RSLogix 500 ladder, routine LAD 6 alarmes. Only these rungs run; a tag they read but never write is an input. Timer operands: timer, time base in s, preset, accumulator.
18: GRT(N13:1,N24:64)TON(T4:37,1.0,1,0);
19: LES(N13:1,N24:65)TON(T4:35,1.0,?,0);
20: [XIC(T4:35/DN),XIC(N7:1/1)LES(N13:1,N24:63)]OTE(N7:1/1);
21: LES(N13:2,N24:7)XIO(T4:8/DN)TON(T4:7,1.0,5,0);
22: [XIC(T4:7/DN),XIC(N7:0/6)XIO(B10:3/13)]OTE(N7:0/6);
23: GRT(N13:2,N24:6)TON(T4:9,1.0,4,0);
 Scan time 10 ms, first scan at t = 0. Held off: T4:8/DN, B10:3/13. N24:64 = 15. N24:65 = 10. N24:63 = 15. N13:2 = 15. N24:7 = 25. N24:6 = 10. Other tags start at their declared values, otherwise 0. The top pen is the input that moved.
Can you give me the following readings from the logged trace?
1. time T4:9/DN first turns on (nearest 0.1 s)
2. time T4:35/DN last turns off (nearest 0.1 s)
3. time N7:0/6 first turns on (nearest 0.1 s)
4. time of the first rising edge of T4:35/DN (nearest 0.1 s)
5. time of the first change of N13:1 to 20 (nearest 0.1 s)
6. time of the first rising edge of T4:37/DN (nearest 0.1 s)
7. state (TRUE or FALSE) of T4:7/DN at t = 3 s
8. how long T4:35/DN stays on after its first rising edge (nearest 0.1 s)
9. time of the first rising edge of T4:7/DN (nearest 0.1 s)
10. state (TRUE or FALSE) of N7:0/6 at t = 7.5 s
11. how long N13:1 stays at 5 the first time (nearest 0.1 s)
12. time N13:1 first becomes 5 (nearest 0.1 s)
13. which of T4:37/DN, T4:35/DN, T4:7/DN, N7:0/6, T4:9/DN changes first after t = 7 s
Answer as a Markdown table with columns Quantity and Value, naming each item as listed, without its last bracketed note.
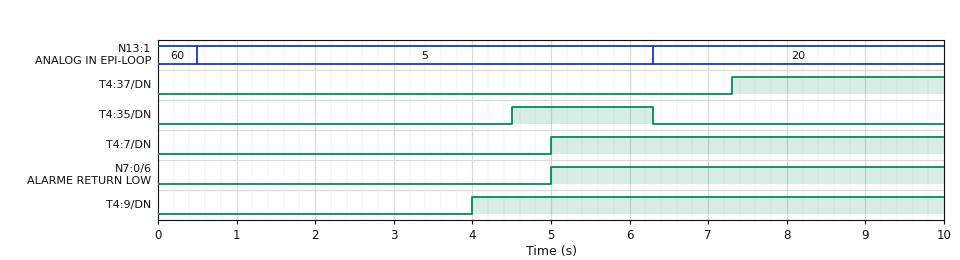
| Quantity | Value |
|---|---|
| time T4:9/DN first turns on | 4.0 s |
| time T4:35/DN last turns off | 6.3 s |
| time N7:0/6 first turns on | 5.0 s |
| time of the first rising edge of T4:35/DN | 4.5 s |
| time of the first change of N13:1 to 20 | 6.3 s |
| time of the first rising edge of T4:37/DN | 7.3 s |
| state (TRUE or FALSE) of T4:7/DN at t = 3 s | FALSE |
| how long T4:35/DN stays on after its first rising edge | 1.8 s |
| time of the first rising edge of T4:7/DN | 5.0 s |
| state (TRUE or FALSE) of N7:0/6 at t = 7.5 s | TRUE |
| how long N13:1 stays at 5 the first time | 5.8 s |
| time N13:1 first becomes 5 | 0.5 s |
| which of T4:37/DN, T4:35/DN, T4:7/DN, N7:0/6, T4:9/DN changes first after t = 7 s | T4:37/DN |
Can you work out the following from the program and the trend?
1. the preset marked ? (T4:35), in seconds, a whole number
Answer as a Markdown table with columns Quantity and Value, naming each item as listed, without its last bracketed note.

| Quantity | Value |
|---|---|
| the preset marked ? (T4:35), in seconds, a whole number | 4 s |
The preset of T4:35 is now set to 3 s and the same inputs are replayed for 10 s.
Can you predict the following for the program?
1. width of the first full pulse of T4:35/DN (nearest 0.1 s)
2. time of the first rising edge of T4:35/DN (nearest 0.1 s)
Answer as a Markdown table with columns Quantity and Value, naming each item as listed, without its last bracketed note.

| Quantity | Value |
|---|---|
| width of the first full pulse of T4:35/DN | 2.8 s |
| time of the first rising edge of T4:35/DN | 3.5 s |
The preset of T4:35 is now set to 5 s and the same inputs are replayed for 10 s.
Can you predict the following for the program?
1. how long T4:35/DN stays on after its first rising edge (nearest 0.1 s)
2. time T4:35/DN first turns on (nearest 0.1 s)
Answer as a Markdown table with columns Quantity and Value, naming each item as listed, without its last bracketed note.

| Quantity | Value |
|---|---|
| how long T4:35/DN stays on after its first rising edge | 0.8 s |
| time T4:35/DN first turns on | 5.5 s |
